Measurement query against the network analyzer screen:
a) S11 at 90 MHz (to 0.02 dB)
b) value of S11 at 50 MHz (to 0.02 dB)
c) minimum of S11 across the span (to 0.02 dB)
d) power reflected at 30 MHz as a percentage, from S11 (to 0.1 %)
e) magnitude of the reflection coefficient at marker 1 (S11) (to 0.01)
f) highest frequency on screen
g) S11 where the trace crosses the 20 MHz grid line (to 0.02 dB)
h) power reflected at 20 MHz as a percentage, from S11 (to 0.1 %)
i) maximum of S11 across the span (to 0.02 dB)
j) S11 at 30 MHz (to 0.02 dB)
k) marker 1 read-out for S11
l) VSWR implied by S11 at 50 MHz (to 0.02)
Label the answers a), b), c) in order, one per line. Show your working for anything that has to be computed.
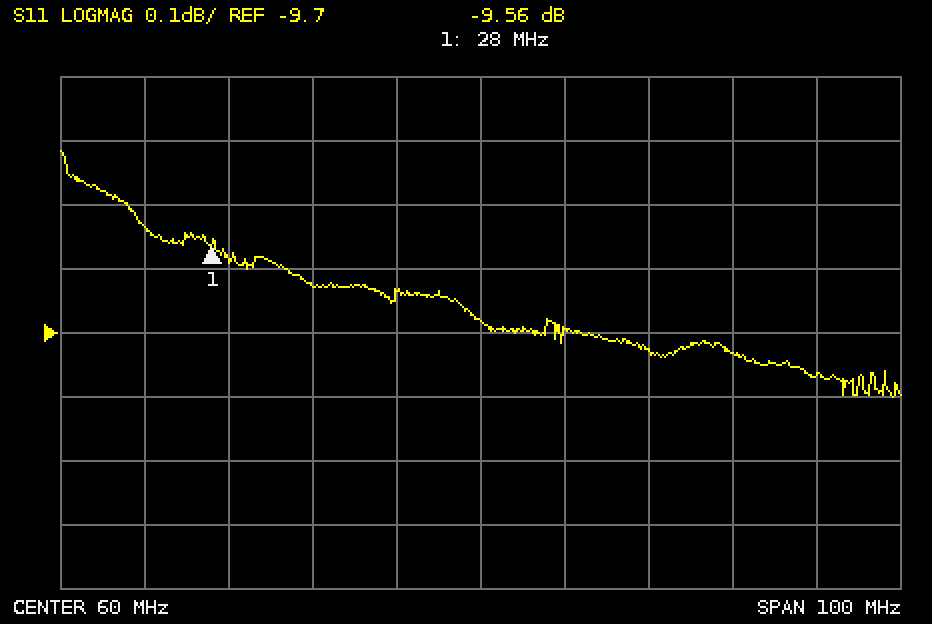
a) -9.74 dB
b) -9.64 dB
c) -9.80 dB
d) 10^(-9.58/10) ≈ 11.0 %
e) 10^(-9.56/20) ≈ 0.33
f) 110 MHz
g) -9.54 dB
h) 10^(-9.54/10) ≈ 11.1 %
i) -9.42 dB
j) -9.58 dB
k) -9.56 dB
l) |Γ| = 10^(-9.64/20) = 0.3296; VSWR = (1 + 0.3296)/(1 − 0.3296) ≈ 1.98
